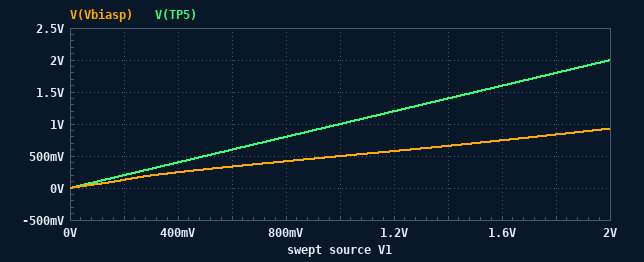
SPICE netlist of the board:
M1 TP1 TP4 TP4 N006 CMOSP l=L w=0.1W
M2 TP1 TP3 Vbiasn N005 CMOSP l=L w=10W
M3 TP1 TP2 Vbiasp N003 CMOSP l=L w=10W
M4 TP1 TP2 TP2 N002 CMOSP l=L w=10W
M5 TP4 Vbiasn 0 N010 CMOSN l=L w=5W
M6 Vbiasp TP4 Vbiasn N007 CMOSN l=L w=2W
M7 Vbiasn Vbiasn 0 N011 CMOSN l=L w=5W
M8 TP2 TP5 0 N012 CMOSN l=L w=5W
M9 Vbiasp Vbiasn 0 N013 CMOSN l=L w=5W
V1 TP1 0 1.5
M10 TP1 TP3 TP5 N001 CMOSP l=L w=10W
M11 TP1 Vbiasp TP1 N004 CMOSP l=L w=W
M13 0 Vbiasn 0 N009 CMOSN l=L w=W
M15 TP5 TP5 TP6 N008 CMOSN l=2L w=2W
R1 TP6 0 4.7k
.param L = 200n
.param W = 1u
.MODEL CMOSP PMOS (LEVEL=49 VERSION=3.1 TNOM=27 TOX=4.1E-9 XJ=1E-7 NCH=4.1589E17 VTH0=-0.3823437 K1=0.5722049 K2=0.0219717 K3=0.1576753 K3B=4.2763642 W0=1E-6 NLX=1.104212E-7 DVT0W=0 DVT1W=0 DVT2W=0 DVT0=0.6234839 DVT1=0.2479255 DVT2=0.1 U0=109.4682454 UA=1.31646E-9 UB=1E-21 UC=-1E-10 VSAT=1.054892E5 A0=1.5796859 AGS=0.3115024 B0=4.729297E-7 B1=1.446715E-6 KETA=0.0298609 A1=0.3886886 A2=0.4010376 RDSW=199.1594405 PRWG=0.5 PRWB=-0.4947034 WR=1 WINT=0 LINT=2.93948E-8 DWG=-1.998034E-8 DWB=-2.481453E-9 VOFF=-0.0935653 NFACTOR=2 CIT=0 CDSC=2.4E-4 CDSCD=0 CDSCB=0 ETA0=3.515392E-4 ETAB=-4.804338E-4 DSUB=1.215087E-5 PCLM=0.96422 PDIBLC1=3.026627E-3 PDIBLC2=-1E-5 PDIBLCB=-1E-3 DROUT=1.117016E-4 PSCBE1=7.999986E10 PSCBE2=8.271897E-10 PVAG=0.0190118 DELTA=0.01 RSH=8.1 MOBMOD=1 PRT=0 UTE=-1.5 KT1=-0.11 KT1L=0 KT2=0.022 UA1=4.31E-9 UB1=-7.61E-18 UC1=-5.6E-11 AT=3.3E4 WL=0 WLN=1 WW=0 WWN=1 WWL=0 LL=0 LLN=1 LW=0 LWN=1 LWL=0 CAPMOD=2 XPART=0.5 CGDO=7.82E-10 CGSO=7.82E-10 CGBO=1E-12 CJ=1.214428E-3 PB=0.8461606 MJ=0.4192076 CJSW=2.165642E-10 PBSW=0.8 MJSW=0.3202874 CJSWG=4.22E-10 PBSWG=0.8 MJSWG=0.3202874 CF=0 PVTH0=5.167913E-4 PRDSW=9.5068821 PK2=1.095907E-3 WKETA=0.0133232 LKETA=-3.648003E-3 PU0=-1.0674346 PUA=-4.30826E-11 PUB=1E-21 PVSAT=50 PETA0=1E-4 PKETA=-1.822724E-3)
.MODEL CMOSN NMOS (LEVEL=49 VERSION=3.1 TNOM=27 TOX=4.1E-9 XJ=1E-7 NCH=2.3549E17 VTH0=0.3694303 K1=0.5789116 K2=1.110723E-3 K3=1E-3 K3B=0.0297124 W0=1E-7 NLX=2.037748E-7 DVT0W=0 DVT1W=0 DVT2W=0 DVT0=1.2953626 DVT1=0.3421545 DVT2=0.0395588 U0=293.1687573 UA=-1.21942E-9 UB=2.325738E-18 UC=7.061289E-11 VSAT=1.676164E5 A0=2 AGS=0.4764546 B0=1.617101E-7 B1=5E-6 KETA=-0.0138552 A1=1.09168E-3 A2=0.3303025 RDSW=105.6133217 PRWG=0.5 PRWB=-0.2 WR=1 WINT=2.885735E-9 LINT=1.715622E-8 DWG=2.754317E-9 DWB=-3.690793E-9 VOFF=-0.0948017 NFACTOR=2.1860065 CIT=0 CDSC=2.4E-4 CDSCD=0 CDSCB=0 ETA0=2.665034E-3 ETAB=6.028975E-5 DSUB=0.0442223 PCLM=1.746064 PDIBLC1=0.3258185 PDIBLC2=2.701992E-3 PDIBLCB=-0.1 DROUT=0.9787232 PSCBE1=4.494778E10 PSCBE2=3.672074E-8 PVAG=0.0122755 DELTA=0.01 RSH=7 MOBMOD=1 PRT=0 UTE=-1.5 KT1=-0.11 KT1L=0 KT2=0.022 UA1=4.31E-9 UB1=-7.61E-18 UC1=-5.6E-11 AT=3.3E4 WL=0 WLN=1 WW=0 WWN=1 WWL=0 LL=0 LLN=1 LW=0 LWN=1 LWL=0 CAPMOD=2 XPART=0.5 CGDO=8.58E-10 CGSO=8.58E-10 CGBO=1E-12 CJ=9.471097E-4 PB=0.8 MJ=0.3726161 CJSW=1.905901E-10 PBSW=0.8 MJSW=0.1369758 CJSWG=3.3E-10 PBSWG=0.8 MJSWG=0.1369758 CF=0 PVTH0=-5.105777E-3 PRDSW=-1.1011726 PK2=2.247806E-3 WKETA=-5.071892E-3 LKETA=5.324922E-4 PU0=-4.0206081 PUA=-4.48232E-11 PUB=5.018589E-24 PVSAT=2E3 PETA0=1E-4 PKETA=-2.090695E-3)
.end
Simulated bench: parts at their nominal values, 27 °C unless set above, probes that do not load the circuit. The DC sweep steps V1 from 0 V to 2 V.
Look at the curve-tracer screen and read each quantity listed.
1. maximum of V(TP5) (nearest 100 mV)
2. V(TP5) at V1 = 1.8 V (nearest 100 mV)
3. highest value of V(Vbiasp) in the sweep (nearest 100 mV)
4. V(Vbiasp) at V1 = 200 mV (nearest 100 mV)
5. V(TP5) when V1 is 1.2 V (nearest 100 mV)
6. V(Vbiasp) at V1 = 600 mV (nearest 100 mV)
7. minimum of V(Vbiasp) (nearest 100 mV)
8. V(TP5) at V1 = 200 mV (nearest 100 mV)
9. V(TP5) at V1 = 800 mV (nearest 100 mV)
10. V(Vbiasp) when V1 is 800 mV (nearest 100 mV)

2.0 V
1.8 V
900 mV
100 mV
1.2 V
300 mV
0 V
200 mV
800 mV
400 mV
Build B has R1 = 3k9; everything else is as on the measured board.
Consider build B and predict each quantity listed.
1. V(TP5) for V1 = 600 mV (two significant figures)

600 mV
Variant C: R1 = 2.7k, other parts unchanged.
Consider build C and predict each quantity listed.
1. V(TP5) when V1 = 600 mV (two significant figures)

600 mV
